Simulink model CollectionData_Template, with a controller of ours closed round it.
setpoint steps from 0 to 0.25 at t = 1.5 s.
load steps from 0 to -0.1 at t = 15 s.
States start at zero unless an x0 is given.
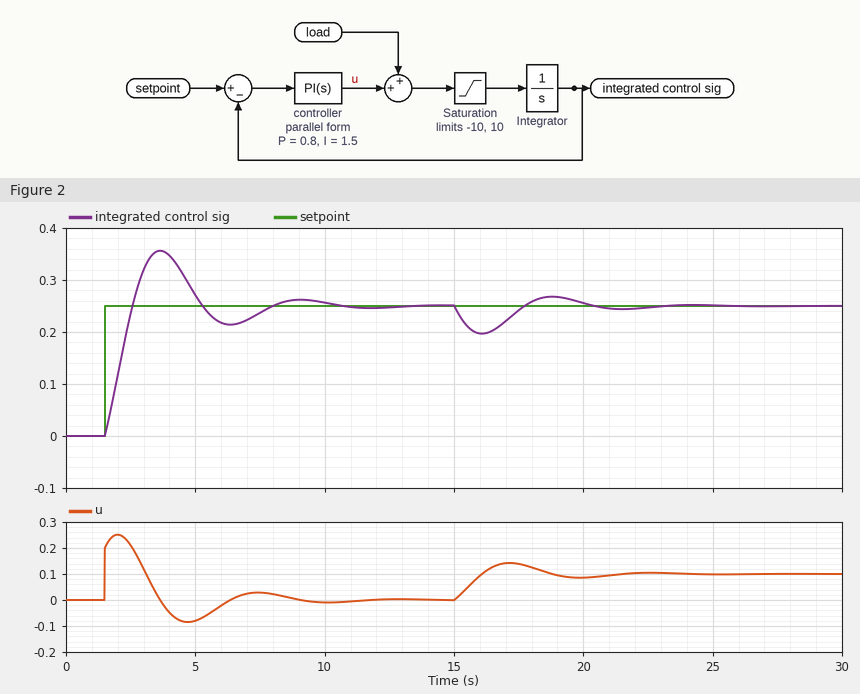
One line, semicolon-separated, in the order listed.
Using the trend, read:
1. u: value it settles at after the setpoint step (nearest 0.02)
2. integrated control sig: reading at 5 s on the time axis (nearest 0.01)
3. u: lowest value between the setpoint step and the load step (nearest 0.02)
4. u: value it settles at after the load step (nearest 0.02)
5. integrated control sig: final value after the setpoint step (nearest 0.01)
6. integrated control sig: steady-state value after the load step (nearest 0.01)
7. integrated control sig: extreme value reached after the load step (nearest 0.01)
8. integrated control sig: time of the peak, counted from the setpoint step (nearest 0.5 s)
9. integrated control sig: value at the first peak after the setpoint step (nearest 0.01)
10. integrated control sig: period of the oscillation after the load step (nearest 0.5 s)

0.00; 0.27; -0.08; 0.10; 0.25; 0.25; 0.20; 2.0 s; 0.36; 5.5 s
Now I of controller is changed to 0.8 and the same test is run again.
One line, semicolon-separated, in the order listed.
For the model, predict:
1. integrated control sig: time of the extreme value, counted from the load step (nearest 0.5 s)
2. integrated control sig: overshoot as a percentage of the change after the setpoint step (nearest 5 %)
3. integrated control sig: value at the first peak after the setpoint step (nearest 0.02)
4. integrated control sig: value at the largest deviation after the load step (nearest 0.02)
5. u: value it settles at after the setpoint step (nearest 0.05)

1.5 s; 35 %; 0.34; 0.18; 0.00
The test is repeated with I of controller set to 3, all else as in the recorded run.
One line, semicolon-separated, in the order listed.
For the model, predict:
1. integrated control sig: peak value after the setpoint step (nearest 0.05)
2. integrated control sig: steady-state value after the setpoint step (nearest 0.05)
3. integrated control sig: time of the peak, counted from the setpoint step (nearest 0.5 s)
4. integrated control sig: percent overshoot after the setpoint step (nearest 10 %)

0.40; 0.25; 1.5 s; 50 %
